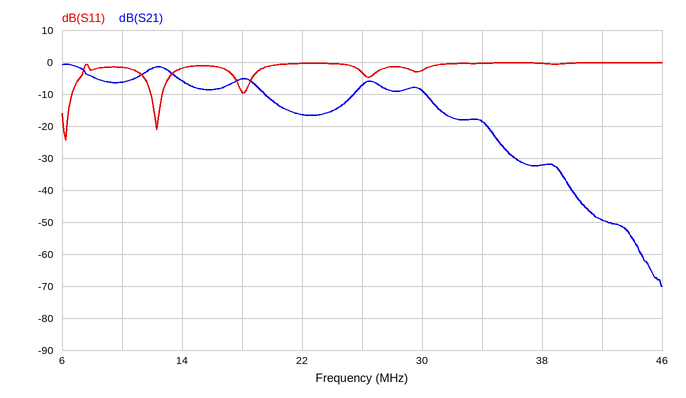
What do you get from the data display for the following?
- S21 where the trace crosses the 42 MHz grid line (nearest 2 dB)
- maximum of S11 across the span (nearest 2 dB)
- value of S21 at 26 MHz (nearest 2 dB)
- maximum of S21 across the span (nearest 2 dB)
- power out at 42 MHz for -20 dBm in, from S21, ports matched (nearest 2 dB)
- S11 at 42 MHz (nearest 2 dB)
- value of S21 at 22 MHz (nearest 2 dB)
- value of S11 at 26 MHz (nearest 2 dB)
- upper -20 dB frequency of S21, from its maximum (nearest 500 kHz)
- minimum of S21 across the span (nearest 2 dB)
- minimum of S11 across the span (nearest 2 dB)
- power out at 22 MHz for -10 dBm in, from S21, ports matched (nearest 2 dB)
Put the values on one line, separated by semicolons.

-50 dB; 0 dB; -8 dB; 0 dB; -70 dBm; 0 dB; -16 dB; -4 dB; 34.5 MHz; -70 dB; -24 dB; -26 dBm
